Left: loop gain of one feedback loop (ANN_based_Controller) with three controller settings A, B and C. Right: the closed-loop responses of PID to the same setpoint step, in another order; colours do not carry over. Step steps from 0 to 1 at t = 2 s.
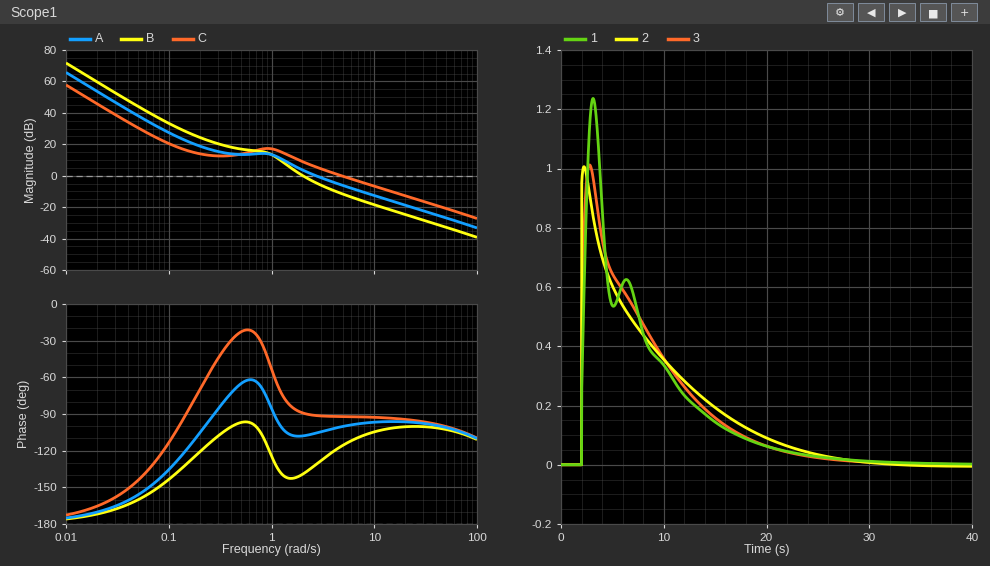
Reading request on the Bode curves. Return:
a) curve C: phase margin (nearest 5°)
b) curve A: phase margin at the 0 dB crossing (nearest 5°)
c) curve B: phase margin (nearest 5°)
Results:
90°
75°
40°
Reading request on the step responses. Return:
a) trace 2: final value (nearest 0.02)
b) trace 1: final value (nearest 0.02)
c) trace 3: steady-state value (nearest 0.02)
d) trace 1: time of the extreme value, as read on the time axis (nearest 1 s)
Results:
0.00
0.00
0.00
3 s
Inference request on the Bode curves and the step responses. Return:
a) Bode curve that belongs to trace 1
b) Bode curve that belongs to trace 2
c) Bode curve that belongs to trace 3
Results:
B
C
A
